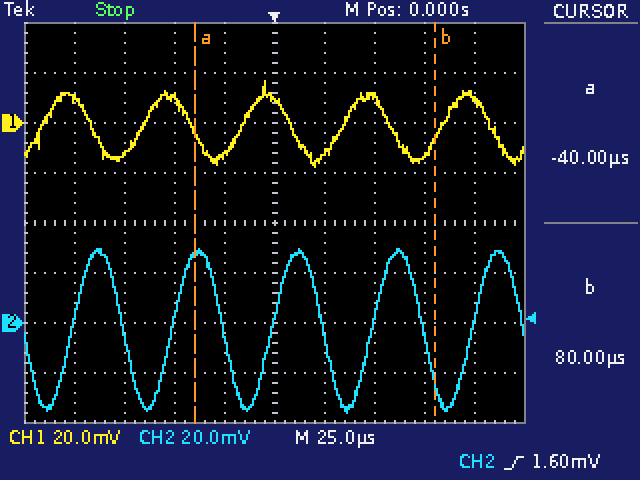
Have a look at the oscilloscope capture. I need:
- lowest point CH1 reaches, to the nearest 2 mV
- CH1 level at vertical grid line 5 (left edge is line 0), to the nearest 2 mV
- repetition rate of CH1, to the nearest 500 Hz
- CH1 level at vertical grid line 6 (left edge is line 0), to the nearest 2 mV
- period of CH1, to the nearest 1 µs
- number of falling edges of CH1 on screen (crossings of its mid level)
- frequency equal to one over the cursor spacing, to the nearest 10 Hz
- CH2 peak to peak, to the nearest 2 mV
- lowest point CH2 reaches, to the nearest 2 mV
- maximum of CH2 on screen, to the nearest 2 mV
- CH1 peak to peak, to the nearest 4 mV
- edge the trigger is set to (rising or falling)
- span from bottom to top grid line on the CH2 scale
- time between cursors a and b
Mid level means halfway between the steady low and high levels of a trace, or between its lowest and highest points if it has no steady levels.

-18 mV
10 mV
20.0 kHz
-12 mV
50 µs
5
8.33 kHz
66 mV
-36 mV
30 mV
36 mV
rising
160 mV
120.0 µs
